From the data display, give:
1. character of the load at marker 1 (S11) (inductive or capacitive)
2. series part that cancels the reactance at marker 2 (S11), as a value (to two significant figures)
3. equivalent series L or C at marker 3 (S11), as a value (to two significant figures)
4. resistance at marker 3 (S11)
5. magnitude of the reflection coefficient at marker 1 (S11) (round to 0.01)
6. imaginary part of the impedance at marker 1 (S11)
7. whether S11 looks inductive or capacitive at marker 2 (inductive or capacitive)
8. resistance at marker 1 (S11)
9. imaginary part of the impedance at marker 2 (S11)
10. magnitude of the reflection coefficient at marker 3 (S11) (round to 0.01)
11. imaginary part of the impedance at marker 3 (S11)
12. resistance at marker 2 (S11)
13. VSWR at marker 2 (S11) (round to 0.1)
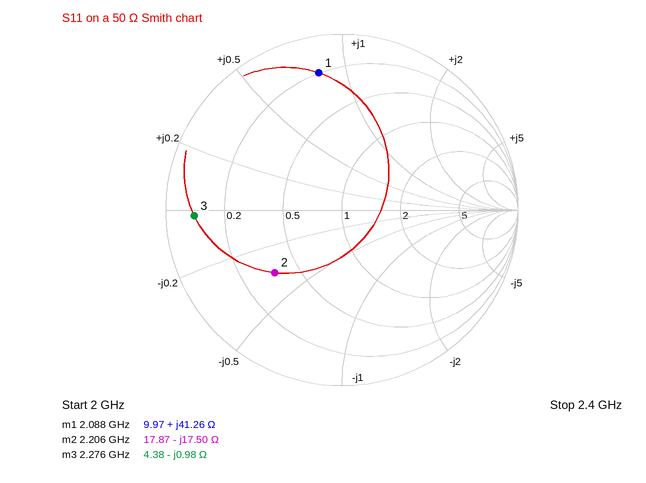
inductive
1.3 nH
71 pF
4.38 Ω
0.79
+41.26 Ω
capacitive
9.97 Ω
-17.50 Ω
0.84
-0.98 Ω
17.87 Ω
3.2
